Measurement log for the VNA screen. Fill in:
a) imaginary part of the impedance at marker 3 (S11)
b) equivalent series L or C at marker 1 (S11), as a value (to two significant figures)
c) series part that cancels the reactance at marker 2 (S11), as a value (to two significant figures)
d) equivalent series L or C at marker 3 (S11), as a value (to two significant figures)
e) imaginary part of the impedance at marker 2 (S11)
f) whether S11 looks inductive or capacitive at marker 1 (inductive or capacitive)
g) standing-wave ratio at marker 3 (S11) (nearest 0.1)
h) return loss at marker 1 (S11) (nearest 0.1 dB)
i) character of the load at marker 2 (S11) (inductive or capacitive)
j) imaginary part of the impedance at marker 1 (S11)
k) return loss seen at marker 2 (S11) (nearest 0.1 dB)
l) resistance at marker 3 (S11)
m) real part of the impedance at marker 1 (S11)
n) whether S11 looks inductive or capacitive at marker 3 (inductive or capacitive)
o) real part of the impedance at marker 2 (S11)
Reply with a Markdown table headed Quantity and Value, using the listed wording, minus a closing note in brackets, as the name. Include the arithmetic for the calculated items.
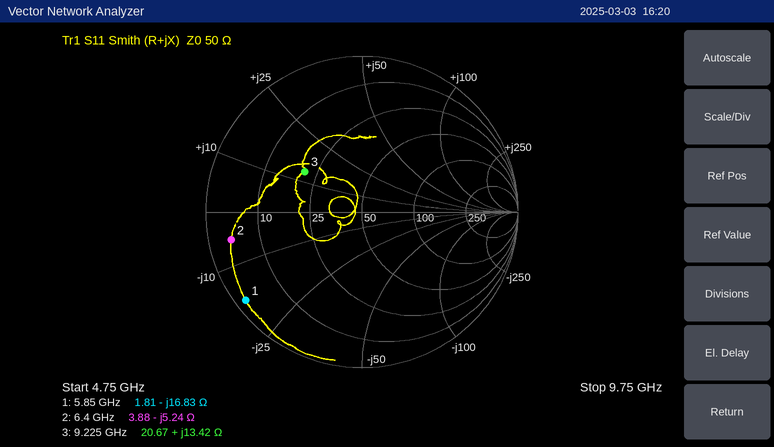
| Quantity | Value |
|---|---|
| imaginary part of the impedance at marker 3 | +13.42 Ω |
| equivalent series L or C at marker 1 (S11), as a value | C = 1/(2π × 5.85 GHz × 16.83 Ω) ≈ 1.6 pF |
| series part that cancels the reactance at marker 2 (S11), as a value | L = 5.24 Ω/(2π × 6.4 GHz) ≈ 130 pH |
| equivalent series L or C at marker 3 (S11), as a value | L = 13.42 Ω/(2π × 9.225 GHz) ≈ 232 pH, so 230 pH to two significant figures |
| imaginary part of the impedance at marker 2 | -5.24 Ω |
| whether S11 looks inductive or capacitive at marker 1 | capacitive |
| standing-wave ratio at marker 3 (S11) | 2.6 |
| return loss at marker 1 (S11) | 0.6 dB |
| character of the load at marker 2 (S11) | capacitive |
| imaginary part of the impedance at marker 1 | -16.83 Ω |
| return loss seen at marker 2 (S11) | 1.3 dB |
| resistance at marker 3 | 20.67 Ω |
| real part of the impedance at marker 1 | 1.81 Ω |
| whether S11 looks inductive or capacitive at marker 3 | inductive |
| real part of the impedance at marker 2 | 3.88 Ω |
